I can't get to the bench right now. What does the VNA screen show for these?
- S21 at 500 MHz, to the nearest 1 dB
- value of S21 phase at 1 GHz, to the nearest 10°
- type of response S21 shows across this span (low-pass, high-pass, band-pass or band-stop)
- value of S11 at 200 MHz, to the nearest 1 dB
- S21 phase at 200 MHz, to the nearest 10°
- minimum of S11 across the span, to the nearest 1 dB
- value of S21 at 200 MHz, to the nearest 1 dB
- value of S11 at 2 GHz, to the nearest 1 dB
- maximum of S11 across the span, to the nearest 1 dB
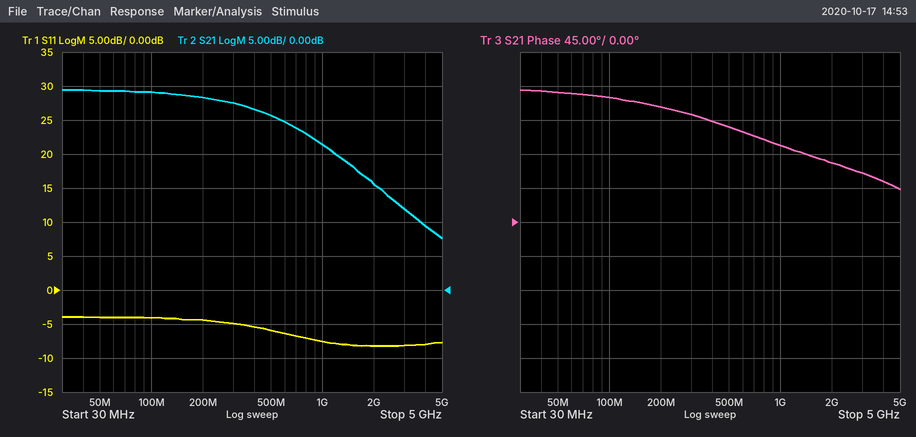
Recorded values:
26 dB
100°
low-pass
-4 dB
150°
-8 dB
28 dB
-8 dB
-4 dB
